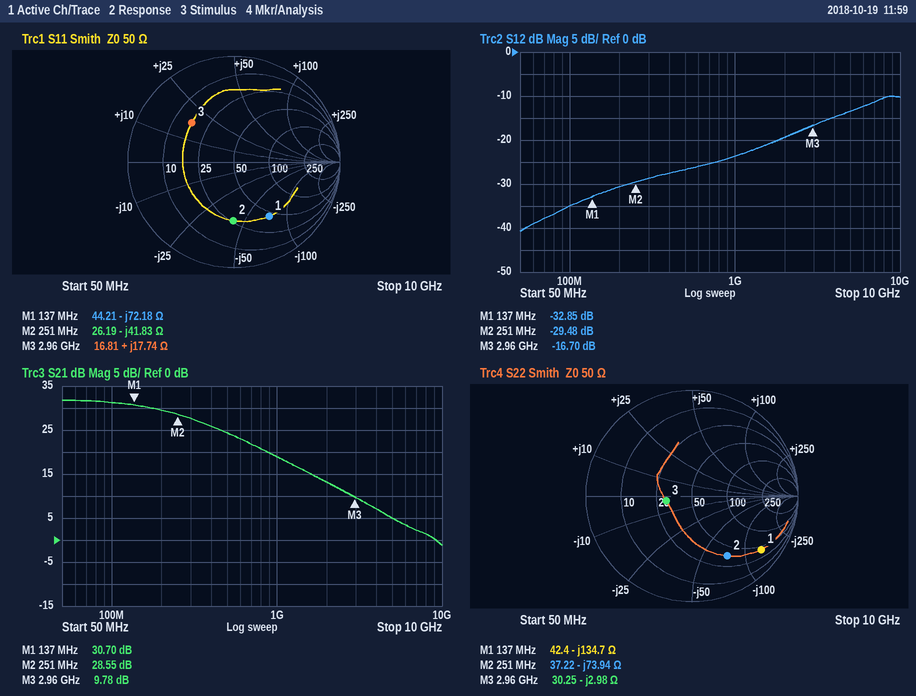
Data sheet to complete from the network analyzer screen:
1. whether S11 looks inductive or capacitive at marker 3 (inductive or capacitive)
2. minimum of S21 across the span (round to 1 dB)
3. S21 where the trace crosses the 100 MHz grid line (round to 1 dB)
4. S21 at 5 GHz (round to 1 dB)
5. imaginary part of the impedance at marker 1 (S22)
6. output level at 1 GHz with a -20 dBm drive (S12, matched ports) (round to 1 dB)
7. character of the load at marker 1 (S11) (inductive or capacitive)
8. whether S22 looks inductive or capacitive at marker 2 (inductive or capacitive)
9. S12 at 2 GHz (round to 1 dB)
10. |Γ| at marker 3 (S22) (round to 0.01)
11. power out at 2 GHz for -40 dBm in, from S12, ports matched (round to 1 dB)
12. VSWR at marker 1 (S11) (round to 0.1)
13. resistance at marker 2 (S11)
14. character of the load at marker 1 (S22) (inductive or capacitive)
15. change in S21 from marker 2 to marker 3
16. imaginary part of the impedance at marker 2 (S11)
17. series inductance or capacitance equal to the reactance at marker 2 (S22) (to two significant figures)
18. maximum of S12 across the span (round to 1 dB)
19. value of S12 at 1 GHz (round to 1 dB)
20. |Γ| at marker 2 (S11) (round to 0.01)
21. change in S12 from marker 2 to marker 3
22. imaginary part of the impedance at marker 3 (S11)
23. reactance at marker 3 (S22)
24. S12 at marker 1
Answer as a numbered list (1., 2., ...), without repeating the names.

1. inductive
2. -1 dB
3. 31 dB
4. 5 dB
5. -134.7 Ω
6. -44 dBm
7. capacitive
8. capacitive
9. -19 dB
10. 0.25
11. -59 dBm
12. 4.1
13. 26.19 Ω
14. capacitive
15. -18.77 dB
16. -41.83 Ω
17. 8.6 pF
18. -10 dB
19. -24 dB
20. 0.55
21. 12.78 dB
22. +17.74 Ω
23. -2.98 Ω
24. -32.85 dB
